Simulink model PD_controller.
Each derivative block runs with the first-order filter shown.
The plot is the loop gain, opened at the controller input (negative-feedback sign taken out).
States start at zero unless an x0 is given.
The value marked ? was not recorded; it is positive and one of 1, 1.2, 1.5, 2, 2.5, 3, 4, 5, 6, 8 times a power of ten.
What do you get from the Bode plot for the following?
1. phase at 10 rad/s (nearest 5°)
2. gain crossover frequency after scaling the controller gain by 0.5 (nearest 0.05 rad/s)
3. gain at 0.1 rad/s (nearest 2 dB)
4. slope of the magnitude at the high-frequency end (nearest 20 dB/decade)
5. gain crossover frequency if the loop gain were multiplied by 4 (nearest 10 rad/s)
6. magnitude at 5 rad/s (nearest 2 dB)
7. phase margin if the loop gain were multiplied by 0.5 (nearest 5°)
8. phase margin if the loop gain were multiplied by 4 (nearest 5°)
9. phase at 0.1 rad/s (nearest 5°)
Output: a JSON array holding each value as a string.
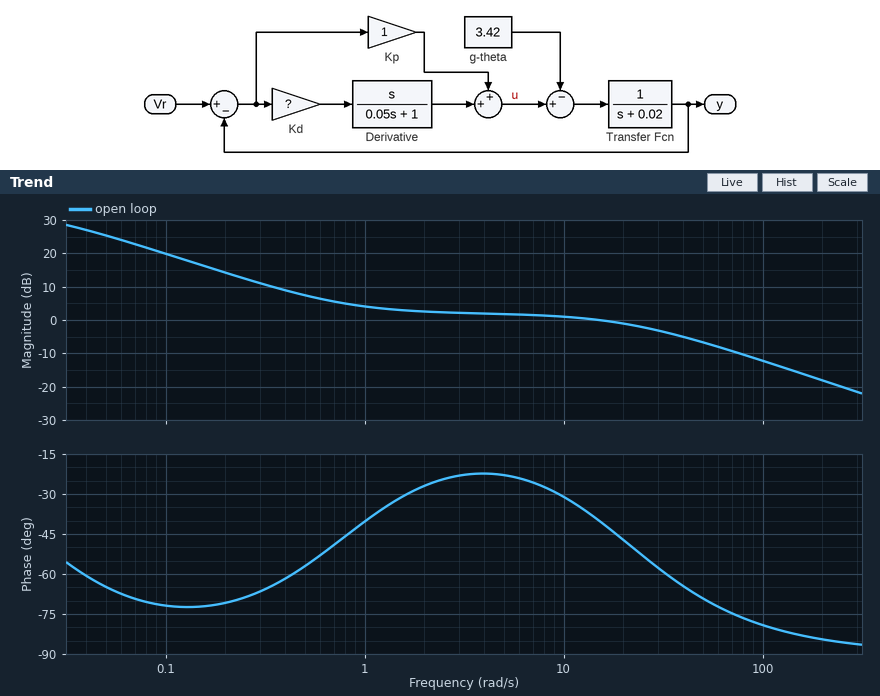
["-30°", "0.65 rad/s", "20 dB", "-20 dB/decade", "100 rad/s", "2 dB", "130°", "100°", "-70°"]
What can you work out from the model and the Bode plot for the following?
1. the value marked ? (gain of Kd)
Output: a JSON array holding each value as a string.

["1.2"]
